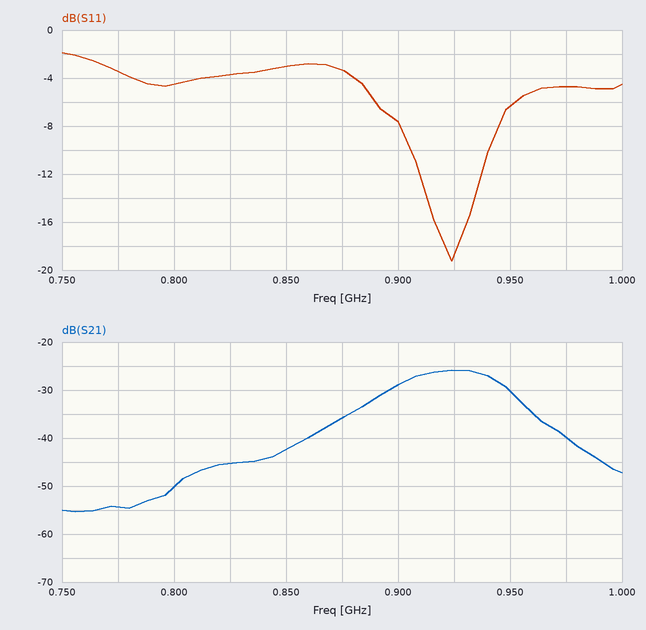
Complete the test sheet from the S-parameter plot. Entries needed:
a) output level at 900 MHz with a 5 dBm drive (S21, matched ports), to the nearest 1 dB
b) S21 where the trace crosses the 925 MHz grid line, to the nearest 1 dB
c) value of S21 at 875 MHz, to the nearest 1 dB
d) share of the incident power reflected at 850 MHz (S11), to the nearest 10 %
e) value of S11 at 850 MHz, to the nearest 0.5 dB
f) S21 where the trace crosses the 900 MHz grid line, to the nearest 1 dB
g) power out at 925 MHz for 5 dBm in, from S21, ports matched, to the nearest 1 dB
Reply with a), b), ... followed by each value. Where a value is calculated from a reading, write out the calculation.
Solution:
a) 5 dBm + (-29 dB) = -24 dBm
b) -26 dB
c) -36 dB
d) 10^(-3/10) ≈ 50 %
e) -3.0 dB
f) -29 dB
g) 5 dBm + (-26 dB) = -21 dBm
